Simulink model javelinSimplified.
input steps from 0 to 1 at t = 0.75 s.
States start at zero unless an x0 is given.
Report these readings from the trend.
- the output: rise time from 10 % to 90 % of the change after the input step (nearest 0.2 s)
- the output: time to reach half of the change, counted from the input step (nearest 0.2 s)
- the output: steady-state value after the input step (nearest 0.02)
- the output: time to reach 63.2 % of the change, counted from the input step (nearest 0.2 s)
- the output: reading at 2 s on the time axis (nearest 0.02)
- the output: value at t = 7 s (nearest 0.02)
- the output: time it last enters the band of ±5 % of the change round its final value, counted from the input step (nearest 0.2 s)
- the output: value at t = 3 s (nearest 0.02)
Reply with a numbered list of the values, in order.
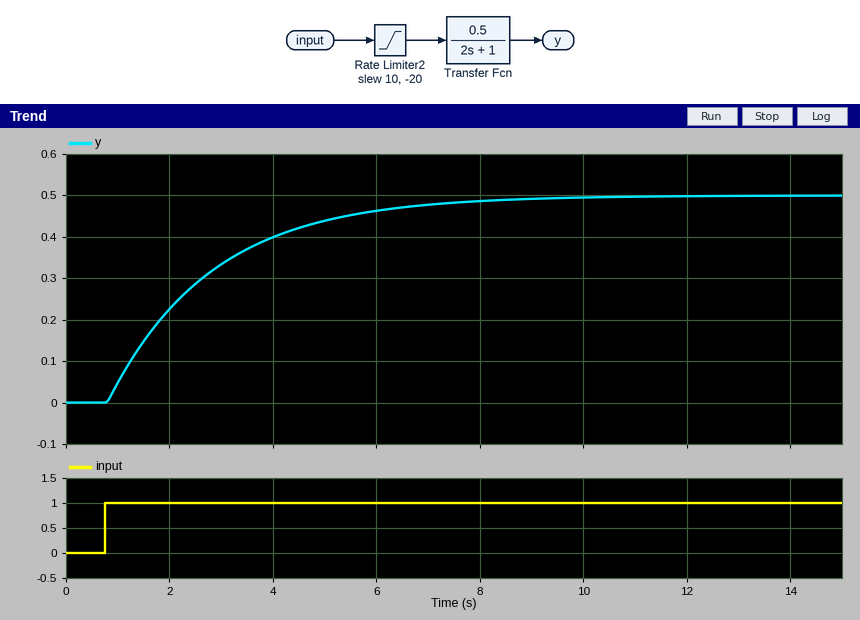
1. 4.4 s
2. 1.4 s
3. 0.50
4. 2.0 s
5. 0.22
6. 0.48
7. 6.0 s
8. 0.34
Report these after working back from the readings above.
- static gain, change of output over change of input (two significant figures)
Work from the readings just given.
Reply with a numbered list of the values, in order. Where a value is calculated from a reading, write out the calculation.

1. (0.5 - 0) / (1 - 0) = 0.50
